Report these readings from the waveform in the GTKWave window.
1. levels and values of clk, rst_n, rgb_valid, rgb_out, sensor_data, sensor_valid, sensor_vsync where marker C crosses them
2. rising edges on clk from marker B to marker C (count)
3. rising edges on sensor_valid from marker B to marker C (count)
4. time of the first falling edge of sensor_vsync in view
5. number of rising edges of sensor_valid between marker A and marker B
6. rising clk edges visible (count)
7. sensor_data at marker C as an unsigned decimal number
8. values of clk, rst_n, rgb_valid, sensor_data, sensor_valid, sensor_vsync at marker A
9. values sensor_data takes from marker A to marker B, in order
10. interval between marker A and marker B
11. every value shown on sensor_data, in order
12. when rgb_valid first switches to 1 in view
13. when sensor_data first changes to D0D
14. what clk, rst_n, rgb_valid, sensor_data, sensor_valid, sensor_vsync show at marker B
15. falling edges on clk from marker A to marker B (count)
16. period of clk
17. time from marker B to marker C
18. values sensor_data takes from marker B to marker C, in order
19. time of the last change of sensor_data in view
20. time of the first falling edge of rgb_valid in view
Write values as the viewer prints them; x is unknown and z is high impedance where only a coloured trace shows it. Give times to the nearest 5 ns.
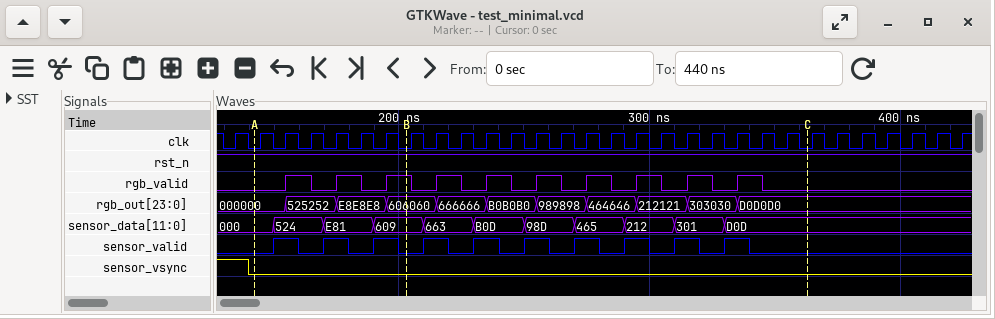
clk=0, rst_n=1, rgb_valid=0, rgb_out=D0D0D0, sensor_data=D0D, sensor_valid=0, sensor_vsync=0
16
7
140 ns
3
30
3341
clk=0, rst_n=1, rgb_valid=0, sensor_data=000, sensor_valid=0, sensor_vsync=0
000, 524, E81, 609
60 ns
000, 524, E81, 609, 663, B0D, 98D, 465, 212, 301, D0D
155 ns
330 ns
clk=0, rst_n=1, rgb_valid=1, sensor_data=609, sensor_valid=0, sensor_vsync=0
6
10 ns
160 ns
609, 663, B0D, 98D, 465, 212, 301, D0D
330 ns
165 ns
